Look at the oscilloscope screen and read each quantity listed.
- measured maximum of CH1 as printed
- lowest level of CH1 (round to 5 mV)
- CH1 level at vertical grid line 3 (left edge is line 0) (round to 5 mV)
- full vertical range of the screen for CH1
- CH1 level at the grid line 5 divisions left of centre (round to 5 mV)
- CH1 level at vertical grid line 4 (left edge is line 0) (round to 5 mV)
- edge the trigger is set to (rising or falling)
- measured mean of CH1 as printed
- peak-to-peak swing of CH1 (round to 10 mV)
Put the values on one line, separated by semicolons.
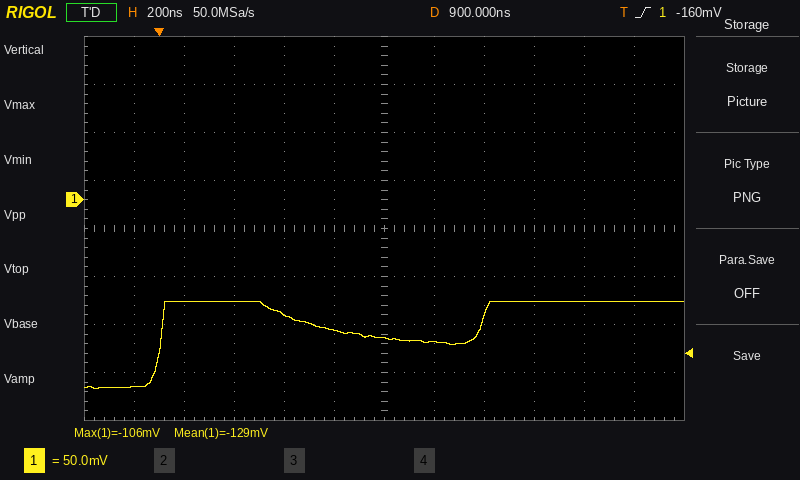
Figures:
-106 mV; -195 mV; -105 mV; 400 mV; -195 mV; -120 mV; rising; -129 mV; 90 mV
